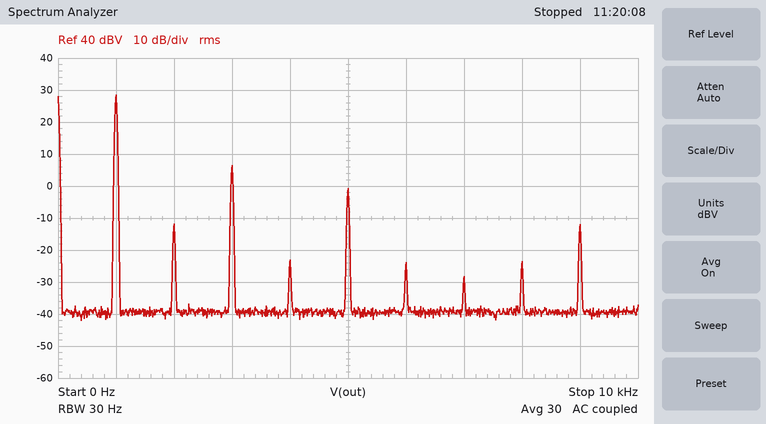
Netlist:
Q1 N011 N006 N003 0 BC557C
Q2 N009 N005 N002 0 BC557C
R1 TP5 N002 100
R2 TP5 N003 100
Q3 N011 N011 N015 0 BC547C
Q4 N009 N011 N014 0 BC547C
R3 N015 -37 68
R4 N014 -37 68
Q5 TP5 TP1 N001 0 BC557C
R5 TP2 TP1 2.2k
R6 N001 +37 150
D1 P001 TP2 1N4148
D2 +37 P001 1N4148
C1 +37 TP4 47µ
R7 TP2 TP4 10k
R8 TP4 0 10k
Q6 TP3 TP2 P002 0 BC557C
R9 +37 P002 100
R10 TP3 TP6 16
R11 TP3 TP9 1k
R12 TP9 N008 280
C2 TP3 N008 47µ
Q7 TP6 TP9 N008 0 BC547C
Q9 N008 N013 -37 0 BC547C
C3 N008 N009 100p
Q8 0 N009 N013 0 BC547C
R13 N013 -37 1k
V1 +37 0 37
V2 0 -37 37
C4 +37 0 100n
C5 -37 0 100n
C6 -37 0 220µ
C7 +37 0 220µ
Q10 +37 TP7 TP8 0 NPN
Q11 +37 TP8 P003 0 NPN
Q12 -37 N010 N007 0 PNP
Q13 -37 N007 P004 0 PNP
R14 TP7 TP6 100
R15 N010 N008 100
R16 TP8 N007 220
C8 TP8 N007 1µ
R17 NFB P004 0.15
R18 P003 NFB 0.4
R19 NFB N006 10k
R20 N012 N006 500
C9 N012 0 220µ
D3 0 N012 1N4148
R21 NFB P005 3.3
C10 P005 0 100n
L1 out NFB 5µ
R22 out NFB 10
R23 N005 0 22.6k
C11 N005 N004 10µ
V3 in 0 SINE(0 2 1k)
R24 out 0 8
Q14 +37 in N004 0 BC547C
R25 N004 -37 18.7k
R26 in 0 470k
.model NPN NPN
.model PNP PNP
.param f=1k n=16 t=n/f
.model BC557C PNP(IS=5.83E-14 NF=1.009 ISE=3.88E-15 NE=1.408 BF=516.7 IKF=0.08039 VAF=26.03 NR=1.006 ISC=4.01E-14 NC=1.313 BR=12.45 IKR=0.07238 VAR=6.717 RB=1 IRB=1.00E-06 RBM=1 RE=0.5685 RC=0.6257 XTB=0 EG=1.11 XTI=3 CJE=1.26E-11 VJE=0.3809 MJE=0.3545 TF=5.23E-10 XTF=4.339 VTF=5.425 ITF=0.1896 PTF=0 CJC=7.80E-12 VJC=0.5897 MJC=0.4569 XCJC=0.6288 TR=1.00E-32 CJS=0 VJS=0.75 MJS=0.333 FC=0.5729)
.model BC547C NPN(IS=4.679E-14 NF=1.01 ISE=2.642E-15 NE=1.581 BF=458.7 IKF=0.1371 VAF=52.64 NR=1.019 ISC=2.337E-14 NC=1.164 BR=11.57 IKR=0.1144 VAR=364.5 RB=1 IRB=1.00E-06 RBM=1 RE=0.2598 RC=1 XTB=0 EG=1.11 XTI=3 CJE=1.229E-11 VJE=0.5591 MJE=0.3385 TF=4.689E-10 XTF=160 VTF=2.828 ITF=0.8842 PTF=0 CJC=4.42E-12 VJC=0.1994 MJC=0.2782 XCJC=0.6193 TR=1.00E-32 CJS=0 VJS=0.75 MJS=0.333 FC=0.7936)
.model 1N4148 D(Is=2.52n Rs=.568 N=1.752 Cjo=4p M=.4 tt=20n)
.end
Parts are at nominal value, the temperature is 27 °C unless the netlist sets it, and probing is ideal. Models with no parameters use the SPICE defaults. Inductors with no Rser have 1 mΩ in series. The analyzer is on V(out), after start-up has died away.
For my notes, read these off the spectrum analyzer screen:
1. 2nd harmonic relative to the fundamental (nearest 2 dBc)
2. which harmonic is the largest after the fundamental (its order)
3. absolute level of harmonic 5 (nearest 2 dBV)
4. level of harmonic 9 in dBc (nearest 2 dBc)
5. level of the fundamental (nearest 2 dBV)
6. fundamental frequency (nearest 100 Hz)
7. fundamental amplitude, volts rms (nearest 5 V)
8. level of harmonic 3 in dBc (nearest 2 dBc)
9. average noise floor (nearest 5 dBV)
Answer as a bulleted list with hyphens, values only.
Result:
- -40 dBc
- 3
- 0 dBV
- -40 dBc
- 28 dBV
- 1.0 kHz
- 25 V
- -22 dBc
- -40 dBV
